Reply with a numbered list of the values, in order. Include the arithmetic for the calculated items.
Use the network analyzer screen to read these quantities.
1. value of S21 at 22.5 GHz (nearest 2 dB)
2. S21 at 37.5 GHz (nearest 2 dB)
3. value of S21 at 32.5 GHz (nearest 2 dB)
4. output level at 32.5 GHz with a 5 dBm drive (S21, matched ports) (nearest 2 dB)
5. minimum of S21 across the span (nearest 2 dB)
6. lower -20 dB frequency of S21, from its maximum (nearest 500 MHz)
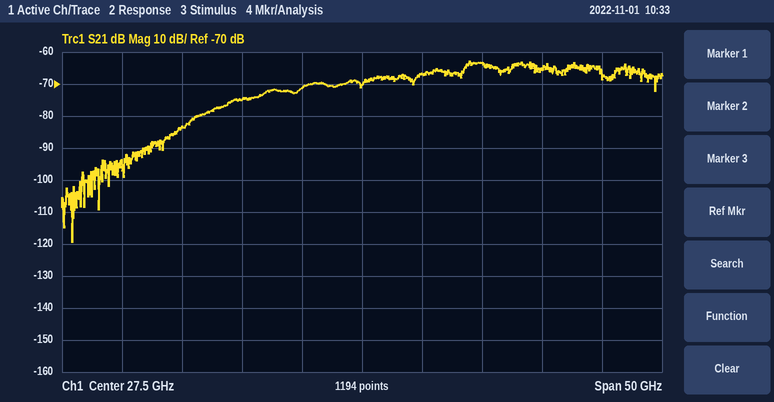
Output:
1. -72 dB
2. -64 dB
3. -66 dB
4. 5 dBm + (-66 dB) = -62 dBm
5. -120 dB
6. 13.0 GHz
